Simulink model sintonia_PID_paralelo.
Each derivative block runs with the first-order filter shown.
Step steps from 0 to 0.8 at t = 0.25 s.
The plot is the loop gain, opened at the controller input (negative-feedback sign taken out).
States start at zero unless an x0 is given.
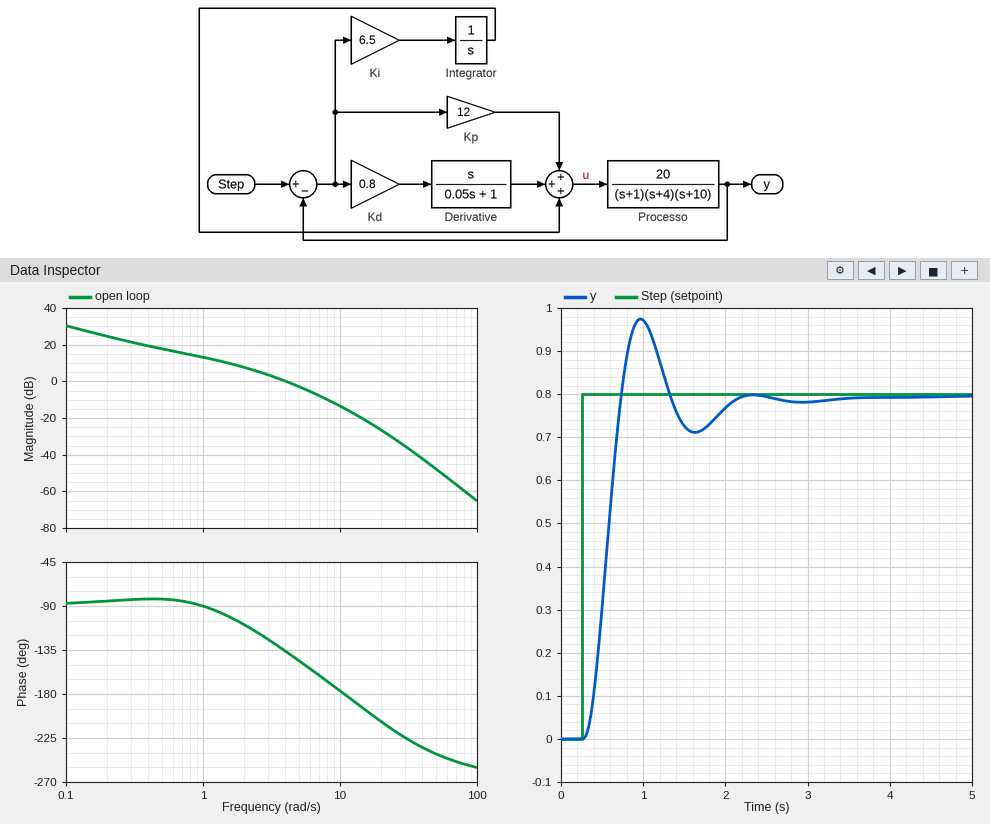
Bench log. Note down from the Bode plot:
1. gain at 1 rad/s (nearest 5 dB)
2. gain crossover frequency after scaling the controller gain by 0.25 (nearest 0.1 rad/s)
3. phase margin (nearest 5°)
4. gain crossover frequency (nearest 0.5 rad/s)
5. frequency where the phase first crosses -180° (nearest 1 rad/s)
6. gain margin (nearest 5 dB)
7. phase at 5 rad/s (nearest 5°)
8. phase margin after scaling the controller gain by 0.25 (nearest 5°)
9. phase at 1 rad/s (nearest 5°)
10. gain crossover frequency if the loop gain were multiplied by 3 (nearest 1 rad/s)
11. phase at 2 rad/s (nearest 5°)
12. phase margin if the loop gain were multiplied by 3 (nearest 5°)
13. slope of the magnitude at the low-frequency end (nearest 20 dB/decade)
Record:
15 dB
1.2 rad/s
45°
4.0 rad/s
11 rad/s
15 dB
-145°
85°
-90°
8 rad/s
-110°
15°
-20 dB/decade
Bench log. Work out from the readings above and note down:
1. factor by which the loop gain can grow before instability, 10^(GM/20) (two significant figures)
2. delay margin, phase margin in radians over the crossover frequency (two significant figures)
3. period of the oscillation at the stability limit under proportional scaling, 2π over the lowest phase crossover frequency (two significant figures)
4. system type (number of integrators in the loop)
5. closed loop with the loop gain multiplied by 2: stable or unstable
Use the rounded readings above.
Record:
5.6
0.20 s
0.57 s
1
stable
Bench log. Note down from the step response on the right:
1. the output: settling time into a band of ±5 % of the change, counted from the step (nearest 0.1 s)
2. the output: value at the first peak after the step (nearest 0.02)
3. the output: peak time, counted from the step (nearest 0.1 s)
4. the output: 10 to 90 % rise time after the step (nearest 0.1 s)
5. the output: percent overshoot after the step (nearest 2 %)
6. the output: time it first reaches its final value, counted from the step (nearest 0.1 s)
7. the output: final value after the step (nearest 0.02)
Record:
1.7 s
0.98
0.7 s
0.3 s
22 %
0.5 s
0.80
